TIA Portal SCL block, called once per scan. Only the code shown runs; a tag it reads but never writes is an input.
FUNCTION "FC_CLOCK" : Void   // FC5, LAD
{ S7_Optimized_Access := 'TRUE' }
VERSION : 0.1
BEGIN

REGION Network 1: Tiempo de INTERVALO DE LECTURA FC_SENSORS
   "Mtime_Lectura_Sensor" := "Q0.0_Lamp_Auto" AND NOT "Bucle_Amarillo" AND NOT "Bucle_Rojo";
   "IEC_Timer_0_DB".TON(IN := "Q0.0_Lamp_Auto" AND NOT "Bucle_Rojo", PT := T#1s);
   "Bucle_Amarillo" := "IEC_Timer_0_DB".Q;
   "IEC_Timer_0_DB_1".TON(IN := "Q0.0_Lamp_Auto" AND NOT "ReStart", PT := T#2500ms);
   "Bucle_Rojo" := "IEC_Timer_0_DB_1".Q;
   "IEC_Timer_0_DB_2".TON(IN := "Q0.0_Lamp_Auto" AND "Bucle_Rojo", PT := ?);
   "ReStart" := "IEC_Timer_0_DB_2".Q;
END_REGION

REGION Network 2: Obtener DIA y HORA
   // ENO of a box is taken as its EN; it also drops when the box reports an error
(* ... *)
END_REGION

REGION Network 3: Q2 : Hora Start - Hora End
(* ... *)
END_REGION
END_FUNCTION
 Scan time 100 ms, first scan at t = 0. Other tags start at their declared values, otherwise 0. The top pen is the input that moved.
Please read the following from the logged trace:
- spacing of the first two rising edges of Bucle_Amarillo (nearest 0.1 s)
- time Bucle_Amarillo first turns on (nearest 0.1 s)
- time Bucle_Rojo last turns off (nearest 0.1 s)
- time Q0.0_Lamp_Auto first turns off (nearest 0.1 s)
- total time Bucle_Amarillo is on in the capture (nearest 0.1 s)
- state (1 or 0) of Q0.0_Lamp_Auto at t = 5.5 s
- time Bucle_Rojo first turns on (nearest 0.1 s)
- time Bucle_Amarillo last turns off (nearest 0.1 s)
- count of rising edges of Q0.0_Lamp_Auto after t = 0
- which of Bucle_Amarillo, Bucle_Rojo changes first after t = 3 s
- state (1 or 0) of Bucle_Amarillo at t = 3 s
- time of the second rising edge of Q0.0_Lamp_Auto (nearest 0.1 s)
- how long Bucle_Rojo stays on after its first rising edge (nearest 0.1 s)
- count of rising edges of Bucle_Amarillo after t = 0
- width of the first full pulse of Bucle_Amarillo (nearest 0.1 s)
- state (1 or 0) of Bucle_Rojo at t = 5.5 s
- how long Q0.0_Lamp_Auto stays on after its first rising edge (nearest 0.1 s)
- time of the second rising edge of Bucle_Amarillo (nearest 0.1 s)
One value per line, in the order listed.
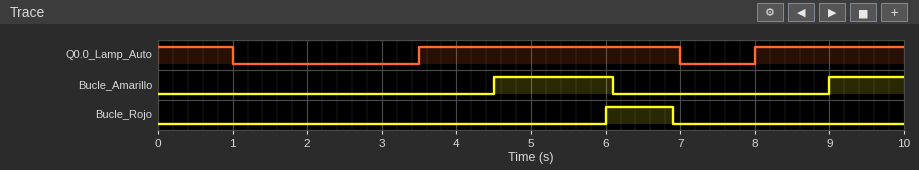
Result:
4.5 s
4.5 s
6.9 s
1.0 s
2.6 s
1
6.0 s
6.1 s
2
Bucle_Amarillo
0
8.0 s
0.9 s
2
1.6 s
0
3.5 s
9.0 s
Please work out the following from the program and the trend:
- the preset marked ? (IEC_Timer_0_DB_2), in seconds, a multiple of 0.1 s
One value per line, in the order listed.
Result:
0.8 s
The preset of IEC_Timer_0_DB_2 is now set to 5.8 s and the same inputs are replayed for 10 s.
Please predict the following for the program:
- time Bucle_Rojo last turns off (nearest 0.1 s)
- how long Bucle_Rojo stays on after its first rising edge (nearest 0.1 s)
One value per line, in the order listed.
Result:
7.0 s
1.0 s
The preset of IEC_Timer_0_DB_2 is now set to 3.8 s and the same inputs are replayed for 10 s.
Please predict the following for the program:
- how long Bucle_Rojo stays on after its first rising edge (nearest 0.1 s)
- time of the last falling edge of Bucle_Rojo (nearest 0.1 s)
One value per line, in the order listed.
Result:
1.0 s
7.0 s
